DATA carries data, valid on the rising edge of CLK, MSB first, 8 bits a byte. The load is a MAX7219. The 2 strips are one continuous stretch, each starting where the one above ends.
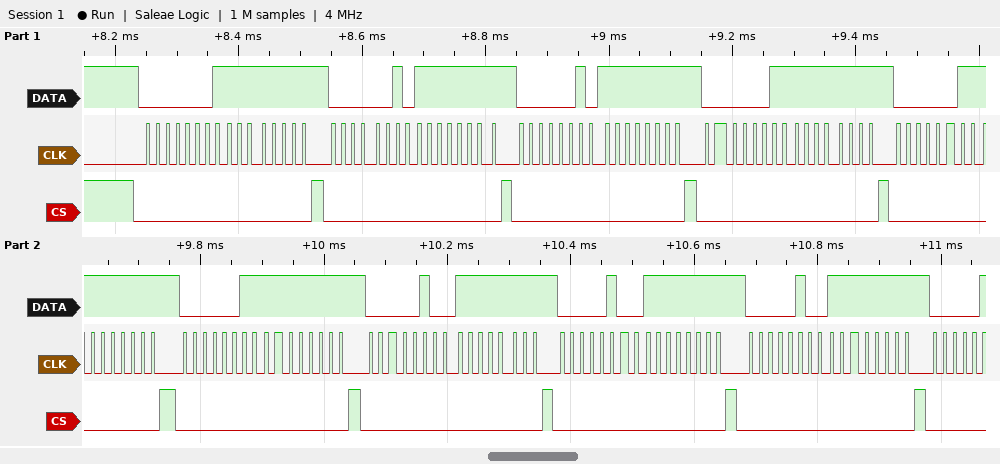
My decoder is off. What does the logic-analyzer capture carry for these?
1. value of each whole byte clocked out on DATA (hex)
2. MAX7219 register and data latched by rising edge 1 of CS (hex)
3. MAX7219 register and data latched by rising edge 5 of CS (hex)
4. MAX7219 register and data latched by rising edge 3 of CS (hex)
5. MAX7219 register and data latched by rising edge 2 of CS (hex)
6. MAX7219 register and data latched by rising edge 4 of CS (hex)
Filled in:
01 FF 02 FF 02 FF 03 FF 03 FF 03 FF 04 FF 04 FF 04 FF
register 0x1, data 0xFF
register 0x3, data 0xFF
register 0x2, data 0xFF
register 0x2, data 0xFF
register 0x3, data 0xFF
